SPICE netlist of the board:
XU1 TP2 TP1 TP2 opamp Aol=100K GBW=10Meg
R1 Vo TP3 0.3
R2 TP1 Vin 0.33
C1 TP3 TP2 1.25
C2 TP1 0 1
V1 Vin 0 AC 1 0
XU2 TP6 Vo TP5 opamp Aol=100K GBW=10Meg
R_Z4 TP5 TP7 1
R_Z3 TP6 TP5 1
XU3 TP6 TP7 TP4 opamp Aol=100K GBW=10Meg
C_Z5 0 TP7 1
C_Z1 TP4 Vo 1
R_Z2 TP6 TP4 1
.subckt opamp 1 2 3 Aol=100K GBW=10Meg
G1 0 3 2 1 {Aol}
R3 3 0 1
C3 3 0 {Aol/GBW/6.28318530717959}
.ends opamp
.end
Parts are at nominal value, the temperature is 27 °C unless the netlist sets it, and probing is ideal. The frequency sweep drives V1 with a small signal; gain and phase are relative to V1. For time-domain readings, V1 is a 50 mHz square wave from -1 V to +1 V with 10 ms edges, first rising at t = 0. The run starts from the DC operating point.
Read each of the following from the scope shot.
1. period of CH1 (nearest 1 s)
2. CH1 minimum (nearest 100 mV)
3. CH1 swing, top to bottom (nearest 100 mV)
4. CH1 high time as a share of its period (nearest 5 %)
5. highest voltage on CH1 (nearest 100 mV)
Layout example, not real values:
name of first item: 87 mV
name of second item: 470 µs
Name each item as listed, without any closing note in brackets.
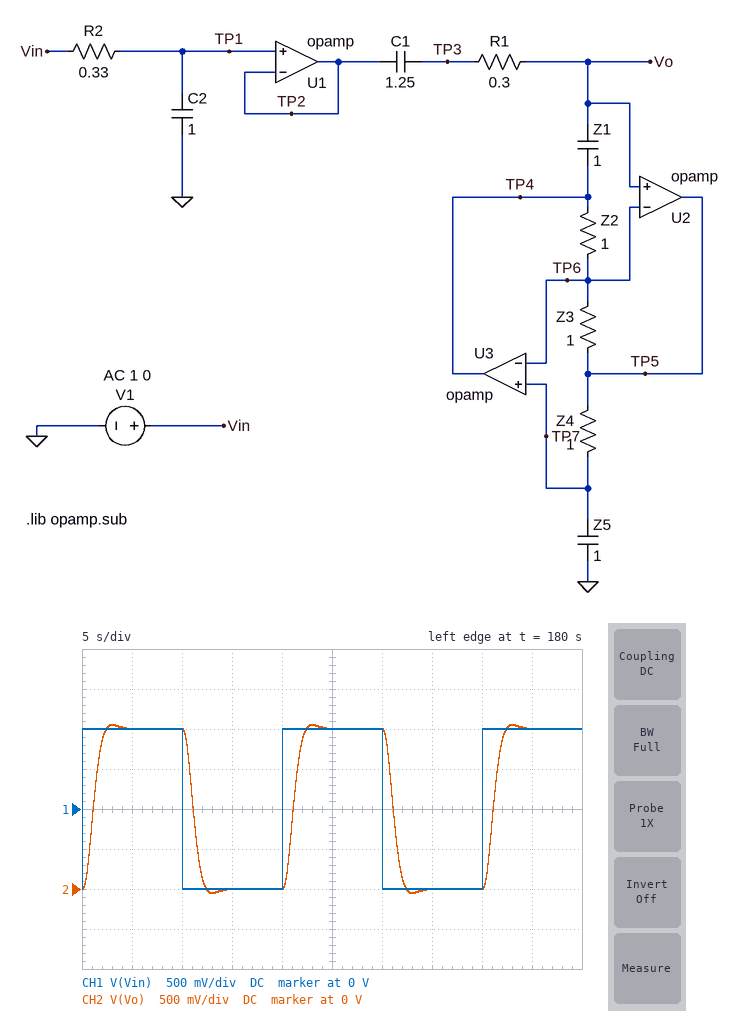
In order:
period of CH1: 20 s
CH1 minimum: -1.0 V
CH1 swing, top to bottom: 2.0 V
CH1 high time as a share of its period: 50 %
highest voltage on CH1: 1.0 V
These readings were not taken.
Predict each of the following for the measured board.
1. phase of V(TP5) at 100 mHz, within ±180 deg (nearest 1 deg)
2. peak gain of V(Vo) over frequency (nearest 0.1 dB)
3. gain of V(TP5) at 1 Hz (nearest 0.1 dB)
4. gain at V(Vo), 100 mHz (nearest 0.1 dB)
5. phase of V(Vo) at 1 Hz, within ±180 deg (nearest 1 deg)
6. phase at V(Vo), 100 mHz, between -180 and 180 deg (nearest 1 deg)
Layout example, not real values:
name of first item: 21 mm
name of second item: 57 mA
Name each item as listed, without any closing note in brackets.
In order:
phase of V(TP5) at 100 mHz, within ±180 deg: -9 deg
peak gain of V(Vo) over frequency: 0 dB
gain of V(TP5) at 1 Hz: -12.7 dB
gain at V(Vo), 100 mHz: -0.3 dB
phase of V(Vo) at 1 Hz, within ±180 deg: 141 deg
phase at V(Vo), 100 mHz, between -180 and 180 deg: -41 deg
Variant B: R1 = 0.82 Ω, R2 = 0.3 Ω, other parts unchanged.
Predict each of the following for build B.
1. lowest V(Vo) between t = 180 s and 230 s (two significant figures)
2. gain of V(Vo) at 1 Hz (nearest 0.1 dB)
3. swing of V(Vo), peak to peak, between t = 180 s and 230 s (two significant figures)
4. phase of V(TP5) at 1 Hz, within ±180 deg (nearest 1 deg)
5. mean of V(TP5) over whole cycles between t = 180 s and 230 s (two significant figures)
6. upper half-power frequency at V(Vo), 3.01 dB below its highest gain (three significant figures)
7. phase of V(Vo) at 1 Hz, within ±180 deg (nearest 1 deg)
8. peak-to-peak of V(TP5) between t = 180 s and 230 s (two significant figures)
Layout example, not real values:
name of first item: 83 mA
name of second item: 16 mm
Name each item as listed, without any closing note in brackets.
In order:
lowest V(Vo) between t = 180 s and 230 s: -400 mV
gain of V(Vo) at 1 Hz: -36.6 dB
swing of V(Vo), peak to peak, between t = 180 s and 230 s: 2.8 V
phase of V(TP5) at 1 Hz, within ±180 deg: -152 deg
mean of V(TP5) over whole cycles between t = 180 s and 230 s: 1.0 V
upper half-power frequency at V(Vo), 3.01 dB below its highest gain: 204 mHz
phase of V(Vo) at 1 Hz, within ±180 deg: 127 deg
peak-to-peak of V(TP5) between t = 180 s and 230 s: 3.5 V
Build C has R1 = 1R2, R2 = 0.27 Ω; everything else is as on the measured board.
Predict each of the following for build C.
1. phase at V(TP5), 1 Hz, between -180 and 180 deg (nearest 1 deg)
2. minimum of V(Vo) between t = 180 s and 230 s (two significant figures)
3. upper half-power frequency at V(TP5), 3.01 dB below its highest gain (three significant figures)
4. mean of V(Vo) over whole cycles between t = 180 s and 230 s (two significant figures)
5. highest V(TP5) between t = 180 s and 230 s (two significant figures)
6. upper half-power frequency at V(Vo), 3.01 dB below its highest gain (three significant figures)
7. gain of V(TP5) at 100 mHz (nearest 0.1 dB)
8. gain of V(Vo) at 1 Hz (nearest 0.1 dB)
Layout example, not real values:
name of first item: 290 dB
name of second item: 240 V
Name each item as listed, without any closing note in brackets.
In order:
phase at V(TP5), 1 Hz, between -180 and 180 deg: -152 deg
minimum of V(Vo) between t = 180 s and 230 s: -570 mV
upper half-power frequency at V(TP5), 3.01 dB below its highest gain: 185 mHz
mean of V(Vo) over whole cycles between t = 180 s and 230 s: 1.0 V
highest V(TP5) between t = 180 s and 230 s: 2.9 V
upper half-power frequency at V(Vo), 3.01 dB below its highest gain: 171 mHz
gain of V(TP5) at 100 mHz: 4.1 dB
gain of V(Vo) at 1 Hz: -39.3 dB
